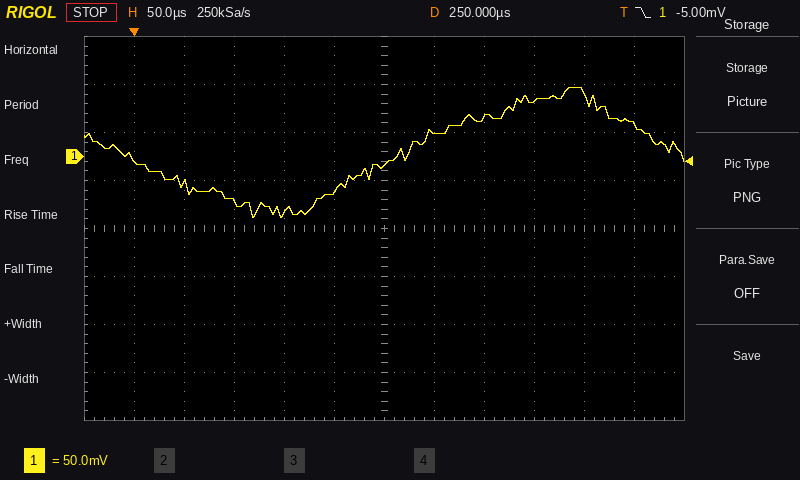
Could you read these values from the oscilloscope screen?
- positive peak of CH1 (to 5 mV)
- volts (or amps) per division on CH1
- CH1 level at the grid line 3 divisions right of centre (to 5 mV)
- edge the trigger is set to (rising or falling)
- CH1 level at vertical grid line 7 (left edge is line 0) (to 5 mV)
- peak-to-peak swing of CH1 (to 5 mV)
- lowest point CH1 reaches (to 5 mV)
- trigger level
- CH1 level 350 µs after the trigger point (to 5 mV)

70 mV
50 mV
60 mV
falling
25 mV
135 mV
-65 mV
-5.00 mV
40 mV
